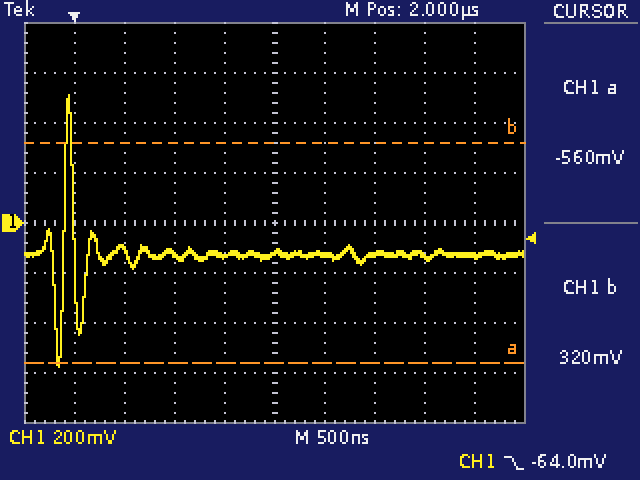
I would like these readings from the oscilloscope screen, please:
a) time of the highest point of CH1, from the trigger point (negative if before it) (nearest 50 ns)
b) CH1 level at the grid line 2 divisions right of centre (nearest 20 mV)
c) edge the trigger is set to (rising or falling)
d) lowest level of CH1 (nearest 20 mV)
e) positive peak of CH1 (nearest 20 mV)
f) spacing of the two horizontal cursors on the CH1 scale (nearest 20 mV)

-50 ns
-120 mV
falling
-580 mV
520 mV
880 mV
